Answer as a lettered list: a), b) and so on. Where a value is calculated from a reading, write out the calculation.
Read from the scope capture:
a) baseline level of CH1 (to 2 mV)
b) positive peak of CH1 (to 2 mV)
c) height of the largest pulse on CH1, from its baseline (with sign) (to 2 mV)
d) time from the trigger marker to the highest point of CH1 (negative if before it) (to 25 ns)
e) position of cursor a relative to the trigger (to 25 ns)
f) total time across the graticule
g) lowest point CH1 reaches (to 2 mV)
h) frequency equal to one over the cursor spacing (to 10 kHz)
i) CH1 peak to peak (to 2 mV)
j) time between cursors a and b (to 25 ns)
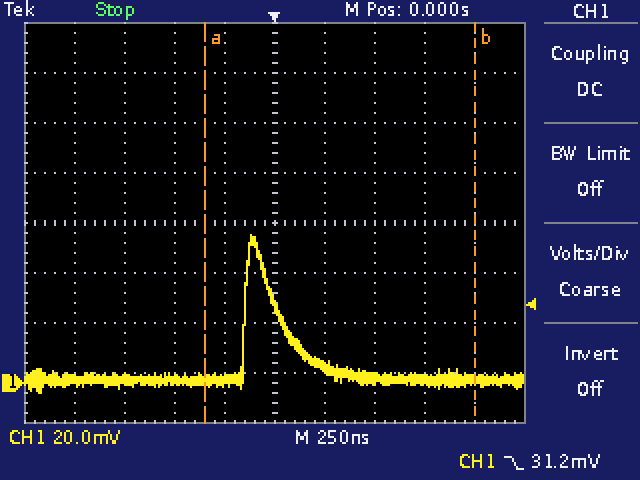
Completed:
a) 2 mV
b) 60 mV
c) 60 mV − (2 mV) = +58 mV
d) -100 ns
e) -350 ns
f) 2.5 µs
g) -4 mV
h) 1 / 1.350 µs ≈ 740 kHz
i) 60 mV − (-4 mV) = 64 mV
j) 1.350 µs
